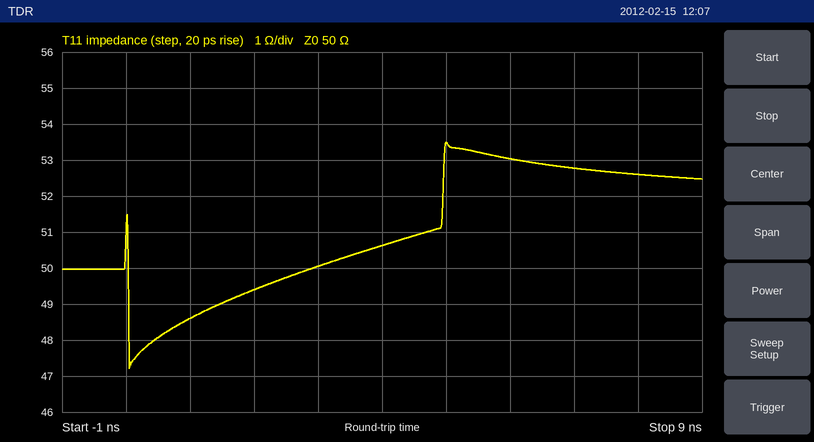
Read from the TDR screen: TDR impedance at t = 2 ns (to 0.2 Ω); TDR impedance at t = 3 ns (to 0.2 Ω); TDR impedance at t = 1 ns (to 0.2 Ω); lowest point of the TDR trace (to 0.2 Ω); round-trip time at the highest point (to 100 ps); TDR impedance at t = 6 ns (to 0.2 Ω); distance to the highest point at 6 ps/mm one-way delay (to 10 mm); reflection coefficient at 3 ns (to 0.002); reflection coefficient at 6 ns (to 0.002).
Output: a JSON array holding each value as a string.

["49.4 Ω", "50.0 Ω", "48.6 Ω", "47.2 Ω", "5.0 ns", "53.0 Ω", "420 mm", "0.000", "+0.030"]
